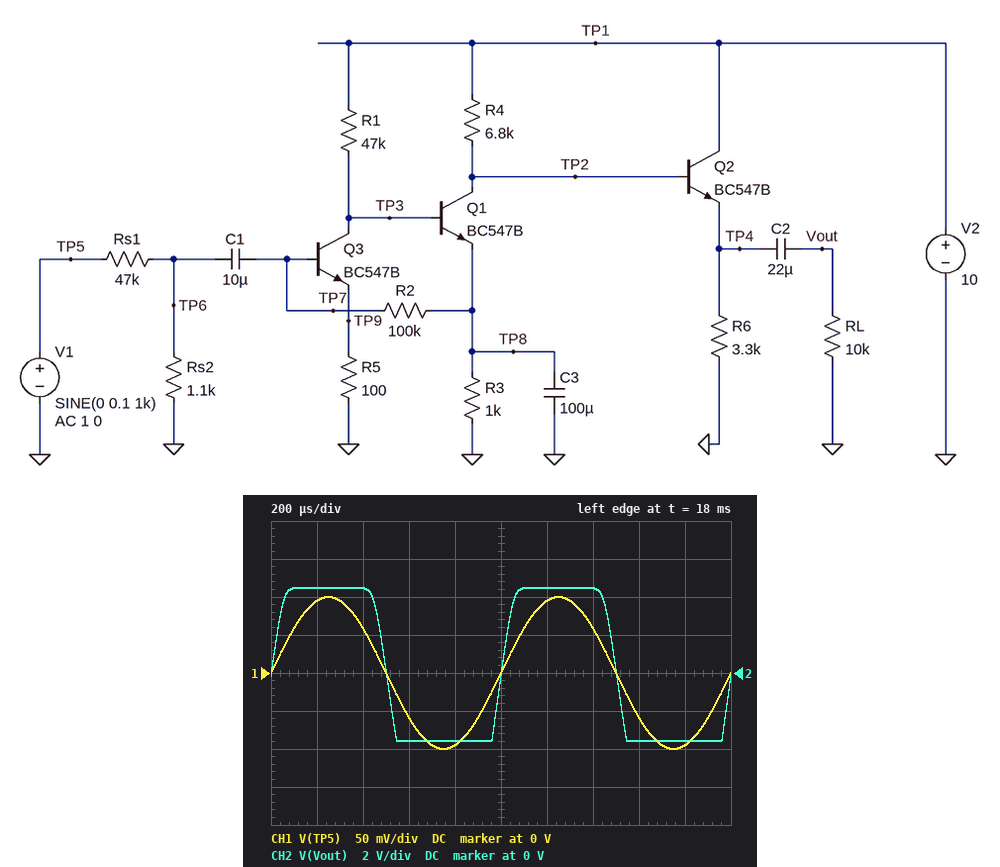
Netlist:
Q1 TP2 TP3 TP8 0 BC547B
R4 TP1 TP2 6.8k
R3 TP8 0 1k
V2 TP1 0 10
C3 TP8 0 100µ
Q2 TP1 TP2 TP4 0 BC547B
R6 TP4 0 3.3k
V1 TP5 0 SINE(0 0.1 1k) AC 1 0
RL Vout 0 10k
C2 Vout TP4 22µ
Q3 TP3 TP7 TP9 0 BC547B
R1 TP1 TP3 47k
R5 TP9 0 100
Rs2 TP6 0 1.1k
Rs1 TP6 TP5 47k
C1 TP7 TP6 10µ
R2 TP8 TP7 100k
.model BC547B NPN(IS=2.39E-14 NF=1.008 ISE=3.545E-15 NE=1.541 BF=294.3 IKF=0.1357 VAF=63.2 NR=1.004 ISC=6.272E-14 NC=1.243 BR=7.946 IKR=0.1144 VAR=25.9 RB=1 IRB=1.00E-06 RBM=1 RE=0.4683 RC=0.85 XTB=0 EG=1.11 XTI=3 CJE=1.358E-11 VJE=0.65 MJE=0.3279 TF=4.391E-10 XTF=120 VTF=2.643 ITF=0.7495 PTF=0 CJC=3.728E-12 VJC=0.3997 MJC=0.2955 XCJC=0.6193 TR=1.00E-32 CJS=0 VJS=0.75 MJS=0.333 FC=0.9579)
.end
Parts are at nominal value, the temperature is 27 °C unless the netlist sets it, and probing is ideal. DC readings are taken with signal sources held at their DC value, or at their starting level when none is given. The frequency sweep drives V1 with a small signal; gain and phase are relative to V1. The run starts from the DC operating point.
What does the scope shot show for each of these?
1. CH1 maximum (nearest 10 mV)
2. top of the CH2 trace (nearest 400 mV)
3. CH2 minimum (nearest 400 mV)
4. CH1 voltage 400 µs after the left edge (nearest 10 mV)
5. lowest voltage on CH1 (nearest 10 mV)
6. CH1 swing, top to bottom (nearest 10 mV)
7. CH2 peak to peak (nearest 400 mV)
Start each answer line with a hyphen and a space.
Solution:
- 100 mV
- 4.4 V
- -3.6 V
- 60 mV
- -100 mV
- 200 mV
- 8.0 V
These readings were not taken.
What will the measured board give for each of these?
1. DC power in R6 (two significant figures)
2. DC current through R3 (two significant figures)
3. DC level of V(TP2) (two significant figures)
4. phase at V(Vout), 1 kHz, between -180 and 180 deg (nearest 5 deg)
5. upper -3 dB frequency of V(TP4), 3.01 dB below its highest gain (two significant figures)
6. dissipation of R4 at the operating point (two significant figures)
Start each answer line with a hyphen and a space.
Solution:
- 6.8 mW
- 680 µA
- 5.4 V
- 0 deg
- 47 kHz
- 3.1 mW
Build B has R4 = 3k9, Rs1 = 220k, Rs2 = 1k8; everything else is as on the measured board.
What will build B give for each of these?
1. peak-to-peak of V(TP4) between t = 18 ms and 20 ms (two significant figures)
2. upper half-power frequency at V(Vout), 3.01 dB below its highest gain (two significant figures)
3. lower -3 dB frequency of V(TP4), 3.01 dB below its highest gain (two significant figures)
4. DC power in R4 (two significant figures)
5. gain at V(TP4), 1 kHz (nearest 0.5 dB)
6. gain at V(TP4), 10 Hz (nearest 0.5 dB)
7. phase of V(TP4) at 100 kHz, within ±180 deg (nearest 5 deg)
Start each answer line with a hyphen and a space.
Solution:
- 5.1 V
- 72 kHz
- 30 Hz
- 1.8 mW
- 29.0 dB
- 17.5 dB
- -55 deg
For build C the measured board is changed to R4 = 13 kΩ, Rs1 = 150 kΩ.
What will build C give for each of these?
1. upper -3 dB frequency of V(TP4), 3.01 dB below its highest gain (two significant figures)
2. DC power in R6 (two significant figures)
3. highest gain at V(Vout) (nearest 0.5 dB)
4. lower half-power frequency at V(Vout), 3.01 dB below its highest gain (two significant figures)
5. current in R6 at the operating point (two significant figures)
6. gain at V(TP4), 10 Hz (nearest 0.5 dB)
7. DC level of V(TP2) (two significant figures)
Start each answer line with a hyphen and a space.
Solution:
- 15 kHz
- 120 µW
- 37.0 dB
- 16 Hz
- 190 µA
- 29.0 dB
- 1.2 V
